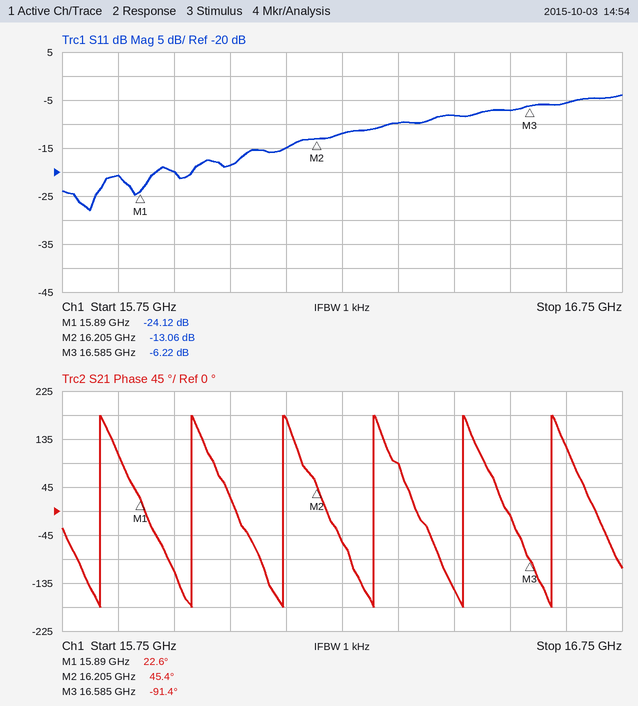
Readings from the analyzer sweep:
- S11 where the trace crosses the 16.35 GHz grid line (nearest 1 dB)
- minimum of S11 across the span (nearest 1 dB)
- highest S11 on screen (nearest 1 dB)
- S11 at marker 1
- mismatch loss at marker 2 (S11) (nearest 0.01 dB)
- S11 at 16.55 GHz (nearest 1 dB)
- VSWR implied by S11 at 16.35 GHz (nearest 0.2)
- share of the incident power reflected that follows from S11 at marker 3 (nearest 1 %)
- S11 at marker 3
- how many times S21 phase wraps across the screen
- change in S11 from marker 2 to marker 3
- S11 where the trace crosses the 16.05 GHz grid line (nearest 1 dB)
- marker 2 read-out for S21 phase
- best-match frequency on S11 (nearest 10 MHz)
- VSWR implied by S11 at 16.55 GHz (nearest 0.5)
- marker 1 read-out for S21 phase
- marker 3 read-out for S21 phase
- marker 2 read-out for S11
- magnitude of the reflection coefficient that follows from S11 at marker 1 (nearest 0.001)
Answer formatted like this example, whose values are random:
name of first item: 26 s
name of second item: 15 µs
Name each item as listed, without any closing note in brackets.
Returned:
S11 where the trace crosses the 16.35 GHz grid line: -10 dB
minimum of S11 across the span: -28 dB
highest S11 on screen: -4 dB
S11 at marker 1: -24.12 dB
mismatch loss at marker 2 (S11): 0.22 dB
S11 at 16.55 GHz: -7 dB
VSWR implied by S11 at 16.35 GHz: 2.0
share of the incident power reflected that follows from S11 at marker 3: 24 %
S11 at marker 3: -6.22 dB
how many times S21 phase wraps across the screen: 6
change in S11 from marker 2 to marker 3: 6.84 dB
S11 where the trace crosses the 16.05 GHz grid line: -19 dB
marker 2 read-out for S21 phase: 45.4°
best-match frequency on S11: 15.80 GHz
VSWR implied by S11 at 16.55 GHz: 2.5
marker 1 read-out for S21 phase: 22.6°
marker 3 read-out for S21 phase: -91.4°
marker 2 read-out for S11: -13.06 dB
magnitude of the reflection coefficient that follows from S11 at marker 1: 0.062
